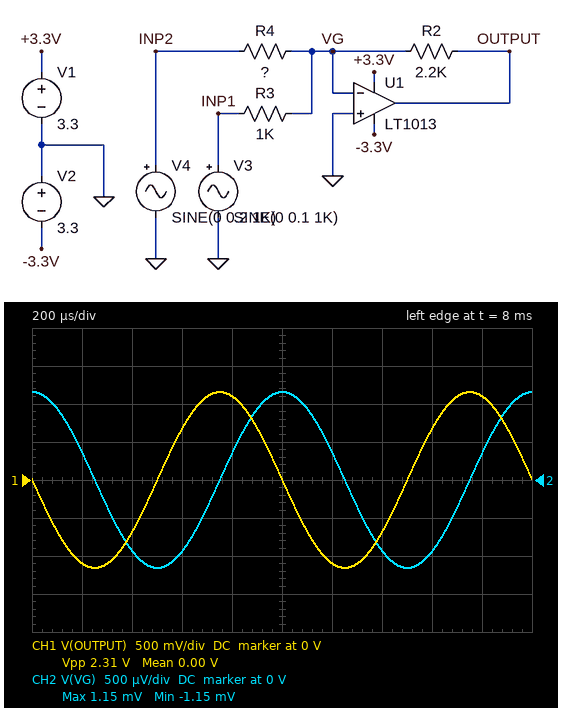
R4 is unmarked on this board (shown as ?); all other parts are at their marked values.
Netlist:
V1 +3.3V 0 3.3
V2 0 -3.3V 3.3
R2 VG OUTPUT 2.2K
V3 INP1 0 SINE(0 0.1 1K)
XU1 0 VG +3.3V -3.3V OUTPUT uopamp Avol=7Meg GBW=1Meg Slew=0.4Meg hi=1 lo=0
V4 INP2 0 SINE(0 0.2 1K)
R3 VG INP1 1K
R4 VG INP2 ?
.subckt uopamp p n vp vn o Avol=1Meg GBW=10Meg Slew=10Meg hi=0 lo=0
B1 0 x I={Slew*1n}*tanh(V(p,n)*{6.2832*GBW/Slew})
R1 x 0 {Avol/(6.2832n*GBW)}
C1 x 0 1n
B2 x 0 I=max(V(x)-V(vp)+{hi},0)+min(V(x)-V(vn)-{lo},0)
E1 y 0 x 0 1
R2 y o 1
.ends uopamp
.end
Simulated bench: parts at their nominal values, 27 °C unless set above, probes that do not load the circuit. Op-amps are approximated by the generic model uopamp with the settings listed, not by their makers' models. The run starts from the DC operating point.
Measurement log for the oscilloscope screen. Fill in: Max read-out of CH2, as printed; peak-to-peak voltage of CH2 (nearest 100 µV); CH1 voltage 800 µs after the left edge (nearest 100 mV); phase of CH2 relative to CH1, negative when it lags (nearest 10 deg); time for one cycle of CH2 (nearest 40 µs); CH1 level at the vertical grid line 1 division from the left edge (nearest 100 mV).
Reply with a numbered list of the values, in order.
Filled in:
1. 1.15 mV
2. 2.3 mV
3. 1.1 V
4. -90 deg
5. 1.00 ms
6. -1.1 V
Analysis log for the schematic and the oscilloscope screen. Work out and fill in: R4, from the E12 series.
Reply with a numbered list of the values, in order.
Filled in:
1. 470 Ω
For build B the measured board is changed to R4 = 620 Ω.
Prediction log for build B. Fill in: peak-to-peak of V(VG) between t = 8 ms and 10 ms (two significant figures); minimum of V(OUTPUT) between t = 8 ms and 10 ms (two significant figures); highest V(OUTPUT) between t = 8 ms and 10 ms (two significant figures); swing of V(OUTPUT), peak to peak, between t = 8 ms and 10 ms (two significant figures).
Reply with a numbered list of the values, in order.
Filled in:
1. 1.9 mV
2. -930 mV
3. 930 mV
4. 1.9 V
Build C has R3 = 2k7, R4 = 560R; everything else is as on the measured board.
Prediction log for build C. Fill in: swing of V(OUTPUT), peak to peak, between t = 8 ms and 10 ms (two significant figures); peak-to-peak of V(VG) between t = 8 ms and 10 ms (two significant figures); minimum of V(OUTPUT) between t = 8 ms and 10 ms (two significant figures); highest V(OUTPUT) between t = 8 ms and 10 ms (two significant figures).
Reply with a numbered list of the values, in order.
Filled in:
1. 1.7 V
2. 1.7 mV
3. -870 mV
4. 870 mV
